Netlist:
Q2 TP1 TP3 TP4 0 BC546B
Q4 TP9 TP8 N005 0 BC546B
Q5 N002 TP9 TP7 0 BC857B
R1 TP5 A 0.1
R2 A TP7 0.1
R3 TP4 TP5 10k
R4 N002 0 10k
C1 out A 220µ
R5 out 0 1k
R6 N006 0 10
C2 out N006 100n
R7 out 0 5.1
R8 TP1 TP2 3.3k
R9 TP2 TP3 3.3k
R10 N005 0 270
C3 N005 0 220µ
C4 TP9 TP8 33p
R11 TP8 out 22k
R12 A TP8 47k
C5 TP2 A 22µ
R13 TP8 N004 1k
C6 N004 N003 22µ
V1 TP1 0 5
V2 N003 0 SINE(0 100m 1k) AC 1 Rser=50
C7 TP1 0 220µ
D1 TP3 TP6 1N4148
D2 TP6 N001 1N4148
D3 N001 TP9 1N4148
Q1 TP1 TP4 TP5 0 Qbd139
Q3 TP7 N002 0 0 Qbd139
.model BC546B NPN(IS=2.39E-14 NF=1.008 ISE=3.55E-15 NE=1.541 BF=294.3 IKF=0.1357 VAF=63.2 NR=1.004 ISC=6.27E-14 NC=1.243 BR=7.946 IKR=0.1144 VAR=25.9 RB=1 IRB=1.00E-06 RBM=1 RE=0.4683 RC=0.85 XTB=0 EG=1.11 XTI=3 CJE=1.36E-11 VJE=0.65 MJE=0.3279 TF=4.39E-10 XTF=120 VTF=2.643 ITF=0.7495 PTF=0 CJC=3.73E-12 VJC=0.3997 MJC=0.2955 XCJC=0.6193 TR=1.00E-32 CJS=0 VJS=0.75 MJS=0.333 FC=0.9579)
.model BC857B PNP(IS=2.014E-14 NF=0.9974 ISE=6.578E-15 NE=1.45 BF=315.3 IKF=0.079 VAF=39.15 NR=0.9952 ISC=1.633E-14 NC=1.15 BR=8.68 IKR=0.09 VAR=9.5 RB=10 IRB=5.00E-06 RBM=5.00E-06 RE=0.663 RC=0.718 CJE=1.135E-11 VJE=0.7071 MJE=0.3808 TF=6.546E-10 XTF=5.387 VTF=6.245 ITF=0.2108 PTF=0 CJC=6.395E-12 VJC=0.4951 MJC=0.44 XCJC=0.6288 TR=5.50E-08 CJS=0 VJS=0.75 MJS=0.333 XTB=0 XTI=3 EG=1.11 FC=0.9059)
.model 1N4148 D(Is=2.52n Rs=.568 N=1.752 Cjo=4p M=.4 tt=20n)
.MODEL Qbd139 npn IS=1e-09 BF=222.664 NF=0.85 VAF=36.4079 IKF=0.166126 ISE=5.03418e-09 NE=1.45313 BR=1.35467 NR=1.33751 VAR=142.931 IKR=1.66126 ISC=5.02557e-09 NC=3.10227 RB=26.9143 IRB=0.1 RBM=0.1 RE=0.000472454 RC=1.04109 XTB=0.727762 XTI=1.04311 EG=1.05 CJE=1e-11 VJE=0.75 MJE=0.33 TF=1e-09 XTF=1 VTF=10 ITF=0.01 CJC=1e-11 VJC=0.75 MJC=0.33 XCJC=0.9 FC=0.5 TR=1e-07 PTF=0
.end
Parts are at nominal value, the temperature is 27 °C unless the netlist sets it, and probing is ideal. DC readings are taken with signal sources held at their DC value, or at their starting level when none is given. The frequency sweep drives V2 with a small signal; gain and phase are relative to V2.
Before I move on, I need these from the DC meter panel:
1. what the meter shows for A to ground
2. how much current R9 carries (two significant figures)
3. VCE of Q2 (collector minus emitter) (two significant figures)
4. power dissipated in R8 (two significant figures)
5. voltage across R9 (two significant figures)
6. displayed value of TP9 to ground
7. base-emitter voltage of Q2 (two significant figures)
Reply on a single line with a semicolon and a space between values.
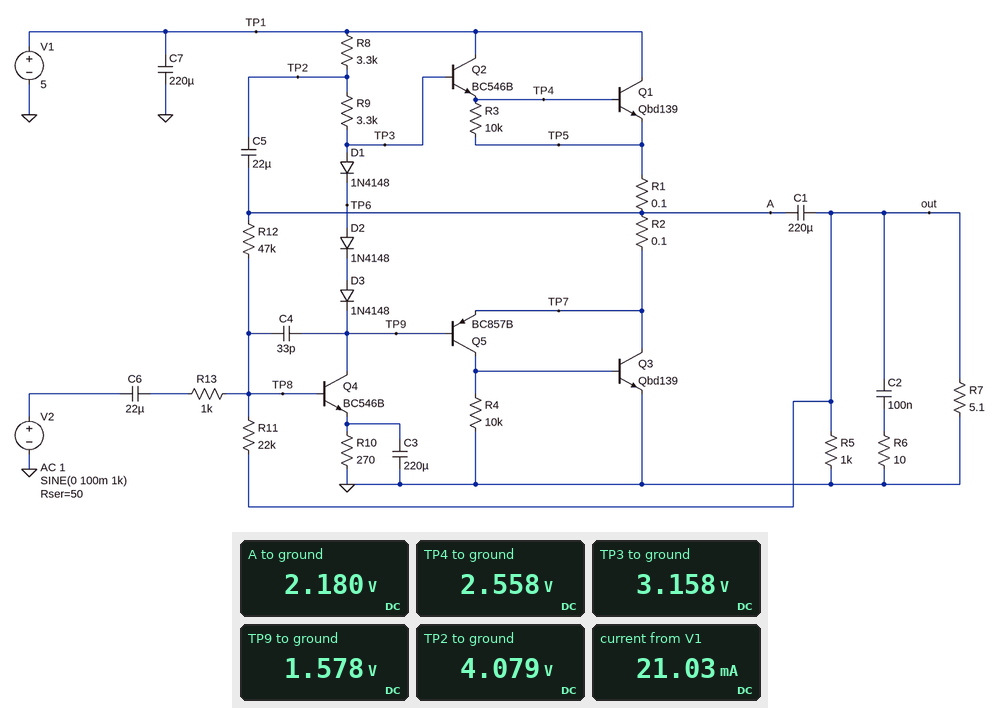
2.180 V; 280 µA; 2.4 V; 260 µW; 920 mV; 1.578 V; 600 mV
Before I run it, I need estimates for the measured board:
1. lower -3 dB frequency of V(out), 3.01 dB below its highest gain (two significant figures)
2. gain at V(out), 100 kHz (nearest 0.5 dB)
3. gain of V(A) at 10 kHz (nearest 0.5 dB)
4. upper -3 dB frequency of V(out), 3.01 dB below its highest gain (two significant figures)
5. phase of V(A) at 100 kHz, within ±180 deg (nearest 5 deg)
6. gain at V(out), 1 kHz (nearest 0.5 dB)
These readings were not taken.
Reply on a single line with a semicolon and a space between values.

43 Hz; 22.0 dB; 22.5 dB; 240 kHz; 155 deg; 22.5 dB
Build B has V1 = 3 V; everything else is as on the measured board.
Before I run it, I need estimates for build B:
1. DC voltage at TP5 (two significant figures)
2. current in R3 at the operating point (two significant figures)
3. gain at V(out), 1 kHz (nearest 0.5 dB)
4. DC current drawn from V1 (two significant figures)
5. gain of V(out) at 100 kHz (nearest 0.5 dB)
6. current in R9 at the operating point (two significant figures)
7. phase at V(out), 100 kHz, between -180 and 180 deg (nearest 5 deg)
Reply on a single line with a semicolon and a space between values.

1.8 V; 26 µA; 4.5 dB; 250 µA; 2.0 dB; 56 µA; 135 deg
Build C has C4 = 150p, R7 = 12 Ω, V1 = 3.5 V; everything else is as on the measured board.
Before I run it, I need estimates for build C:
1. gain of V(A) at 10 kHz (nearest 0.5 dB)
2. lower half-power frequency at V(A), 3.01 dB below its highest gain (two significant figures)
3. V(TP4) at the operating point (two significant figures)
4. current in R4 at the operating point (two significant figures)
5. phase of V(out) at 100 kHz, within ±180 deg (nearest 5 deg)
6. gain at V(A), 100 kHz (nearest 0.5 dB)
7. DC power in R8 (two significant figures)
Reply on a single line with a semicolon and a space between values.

20.5 dB; 7.1 Hz; 2.2 V; 32 µA; 105 deg; 13.0 dB; 37 µW
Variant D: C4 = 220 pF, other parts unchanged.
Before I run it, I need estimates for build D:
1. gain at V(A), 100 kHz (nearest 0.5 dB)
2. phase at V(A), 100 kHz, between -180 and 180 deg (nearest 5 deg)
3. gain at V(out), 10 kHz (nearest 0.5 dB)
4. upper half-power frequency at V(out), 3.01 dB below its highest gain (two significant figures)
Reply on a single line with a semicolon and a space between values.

14.0 dB; 110 deg; 22.0 dB; 41 kHz
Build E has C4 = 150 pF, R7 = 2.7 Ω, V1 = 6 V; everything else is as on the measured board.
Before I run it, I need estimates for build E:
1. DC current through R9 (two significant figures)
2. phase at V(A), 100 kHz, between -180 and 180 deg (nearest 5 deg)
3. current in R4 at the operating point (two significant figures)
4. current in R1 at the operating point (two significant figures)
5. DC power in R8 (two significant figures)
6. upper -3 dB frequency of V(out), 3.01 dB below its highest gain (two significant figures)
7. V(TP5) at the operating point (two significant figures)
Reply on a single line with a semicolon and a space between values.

400 µA; 120 deg; 40 µA; 39 mA; 530 µW; 59 kHz; 2.3 V
